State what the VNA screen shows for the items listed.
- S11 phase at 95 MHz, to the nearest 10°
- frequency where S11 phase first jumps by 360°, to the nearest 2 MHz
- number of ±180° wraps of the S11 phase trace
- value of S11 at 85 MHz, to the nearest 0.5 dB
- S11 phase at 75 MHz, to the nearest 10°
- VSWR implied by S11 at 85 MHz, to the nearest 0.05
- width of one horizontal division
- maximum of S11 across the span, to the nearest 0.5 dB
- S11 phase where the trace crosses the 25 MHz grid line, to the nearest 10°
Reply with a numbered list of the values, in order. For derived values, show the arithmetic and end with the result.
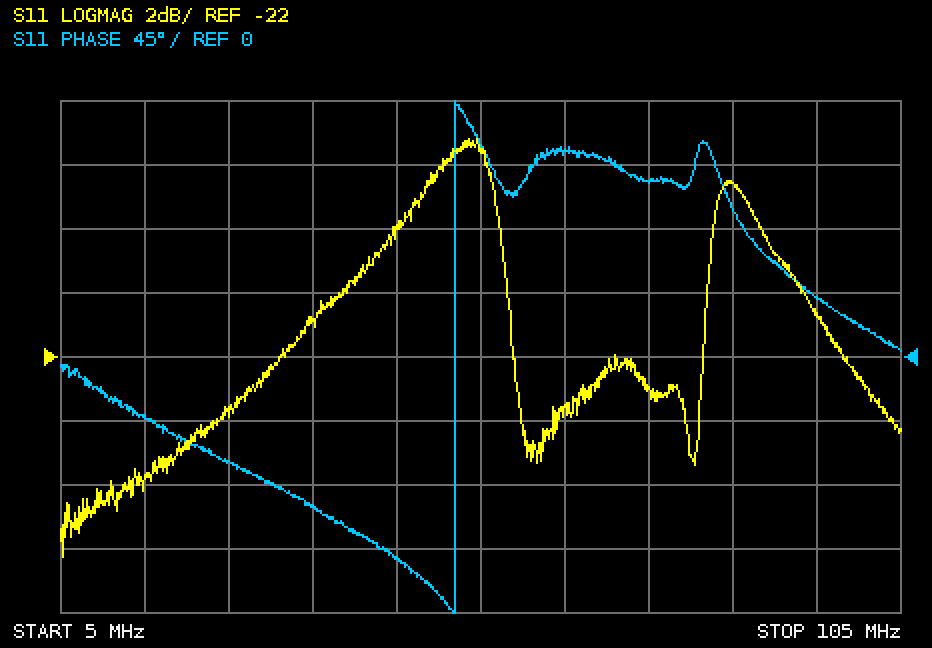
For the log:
1. 40°
2. 52 MHz
3. 1
4. -16.5 dB
5. 120°
6. |Γ| = 10^(-16.5/20) = 0.1496; VSWR = (1 + 0.1496)/(1 − 0.1496) ≈ 1.35
7. 10 MHz
8. -15.0 dB
9. -70°
